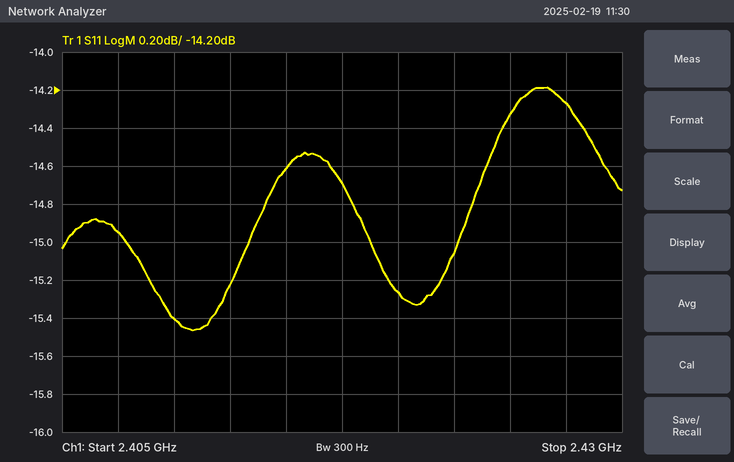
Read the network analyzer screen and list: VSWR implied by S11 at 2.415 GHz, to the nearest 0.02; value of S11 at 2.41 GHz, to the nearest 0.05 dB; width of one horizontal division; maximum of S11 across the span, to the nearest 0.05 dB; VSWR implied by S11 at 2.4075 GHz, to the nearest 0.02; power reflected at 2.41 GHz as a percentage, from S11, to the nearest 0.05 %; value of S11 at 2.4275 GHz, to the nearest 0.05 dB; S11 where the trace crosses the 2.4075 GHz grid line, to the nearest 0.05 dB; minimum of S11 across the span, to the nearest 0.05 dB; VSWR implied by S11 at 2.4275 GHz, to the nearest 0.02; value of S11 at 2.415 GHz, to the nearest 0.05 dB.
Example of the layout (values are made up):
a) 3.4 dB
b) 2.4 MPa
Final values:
a) 1.46
b) -15.40 dB
c) 2.5 MHz
d) -14.20 dB
e) 1.44
f) 2.90 %
g) -14.25 dB
h) -14.95 dB
i) -15.45 dB
j) 1.48
k) -14.60 dB
